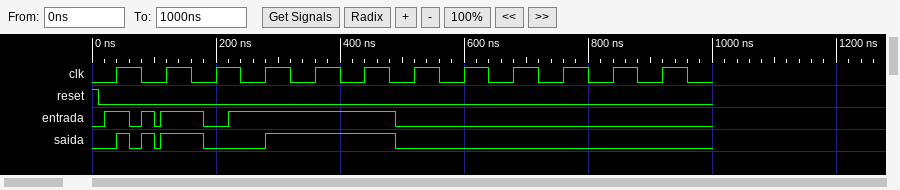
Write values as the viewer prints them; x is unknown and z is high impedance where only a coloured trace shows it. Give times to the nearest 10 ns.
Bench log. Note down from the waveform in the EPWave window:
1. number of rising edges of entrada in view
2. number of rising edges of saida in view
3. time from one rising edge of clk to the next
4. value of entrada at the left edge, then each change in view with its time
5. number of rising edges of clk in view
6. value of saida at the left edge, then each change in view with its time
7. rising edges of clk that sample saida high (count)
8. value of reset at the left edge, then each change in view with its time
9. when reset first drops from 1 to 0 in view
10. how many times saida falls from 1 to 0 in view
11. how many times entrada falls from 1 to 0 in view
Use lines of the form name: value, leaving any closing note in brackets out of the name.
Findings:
number of rising edges of entrada in view: 4
number of rising edges of saida in view: 4
time from one rising edge of clk to the next: 80 ns
value of entrada at the left edge, then each change in view with its time: 0, 1 at 20 ns, 0 at 60 ns, 1 at 80 ns, 0 at 100 ns, 1 at 110 ns, 0 at 180 ns, 1 at 220 ns, 0 at 490 ns
number of rising edges of clk in view: 12
value of saida at the left edge, then each change in view with its time: 0, 1 at 40 ns, 0 at 60 ns, 1 at 80 ns, 0 at 100 ns, 1 at 110 ns, 0 at 180 ns, 1 at 280 ns, 0 at 490 ns
rising edges of clk that sample saida high: 3
value of reset at the left edge, then each change in view with its time: 1, 0 at 10 ns
when reset first drops from 1 to 0 in view: 10 ns
how many times saida falls from 1 to 0 in view: 4
how many times entrada falls from 1 to 0 in view: 4
